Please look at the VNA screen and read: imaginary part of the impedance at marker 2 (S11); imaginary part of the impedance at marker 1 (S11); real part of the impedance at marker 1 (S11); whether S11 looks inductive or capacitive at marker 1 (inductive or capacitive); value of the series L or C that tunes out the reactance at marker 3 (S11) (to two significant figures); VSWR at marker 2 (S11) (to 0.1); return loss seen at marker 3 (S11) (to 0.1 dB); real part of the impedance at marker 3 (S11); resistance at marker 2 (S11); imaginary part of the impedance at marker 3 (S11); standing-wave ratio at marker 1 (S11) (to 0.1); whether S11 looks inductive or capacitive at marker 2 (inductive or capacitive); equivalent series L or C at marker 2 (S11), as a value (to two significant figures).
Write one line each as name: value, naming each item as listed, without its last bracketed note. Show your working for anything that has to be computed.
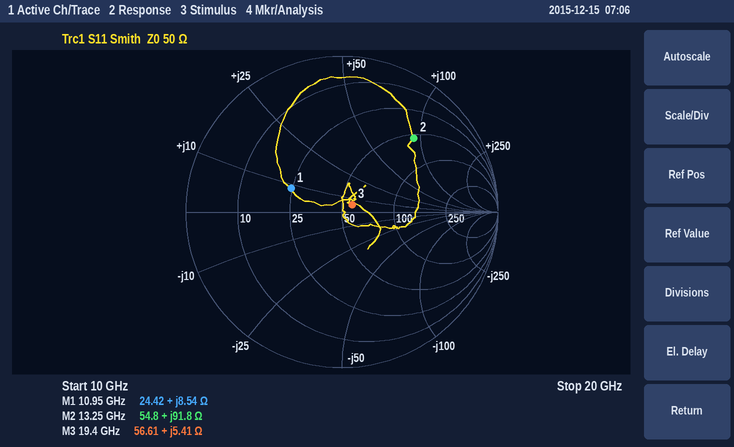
imaginary part of the impedance at marker 2: +91.8 Ω
imaginary part of the impedance at marker 1: +8.54 Ω
real part of the impedance at marker 1: 24.42 Ω
whether S11 looks inductive or capacitive at marker 1: inductive
value of the series L or C that tunes out the reactance at marker 3 (S11): C = 1/(2π × 19.4 GHz × 5.41 Ω) ≈ 1.5 pF
VSWR at marker 2 (S11): 4.9
return loss seen at marker 3 (S11): 21.9 dB
real part of the impedance at marker 3: 56.61 Ω
resistance at marker 2: 54.8 Ω
imaginary part of the impedance at marker 3: +5.41 Ω
standing-wave ratio at marker 1 (S11): 2.1
whether S11 looks inductive or capacitive at marker 2: inductive
equivalent series L or C at marker 2 (S11), as a value: L = 91.8 Ω/(2π × 13.25 GHz) ≈ 1.1 nH
